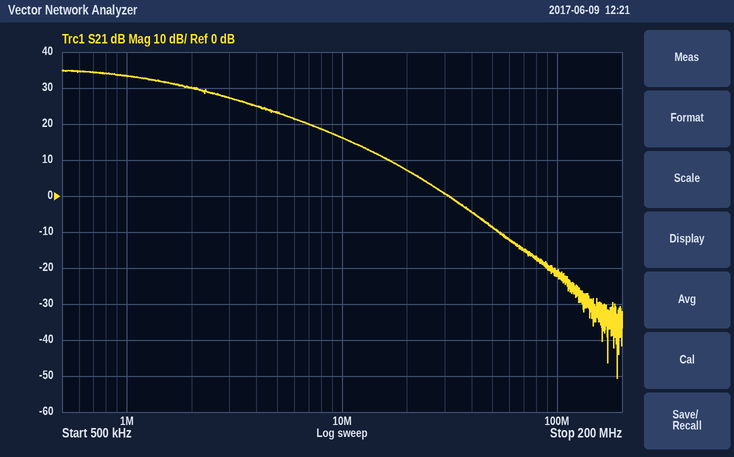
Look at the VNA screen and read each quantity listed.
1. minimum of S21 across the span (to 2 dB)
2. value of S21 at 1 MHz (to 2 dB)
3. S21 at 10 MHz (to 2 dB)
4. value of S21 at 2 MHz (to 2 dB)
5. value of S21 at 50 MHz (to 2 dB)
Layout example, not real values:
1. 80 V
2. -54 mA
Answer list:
1. -50 dB
2. 34 dB
3. 16 dB
4. 30 dB
5. -8 dB
